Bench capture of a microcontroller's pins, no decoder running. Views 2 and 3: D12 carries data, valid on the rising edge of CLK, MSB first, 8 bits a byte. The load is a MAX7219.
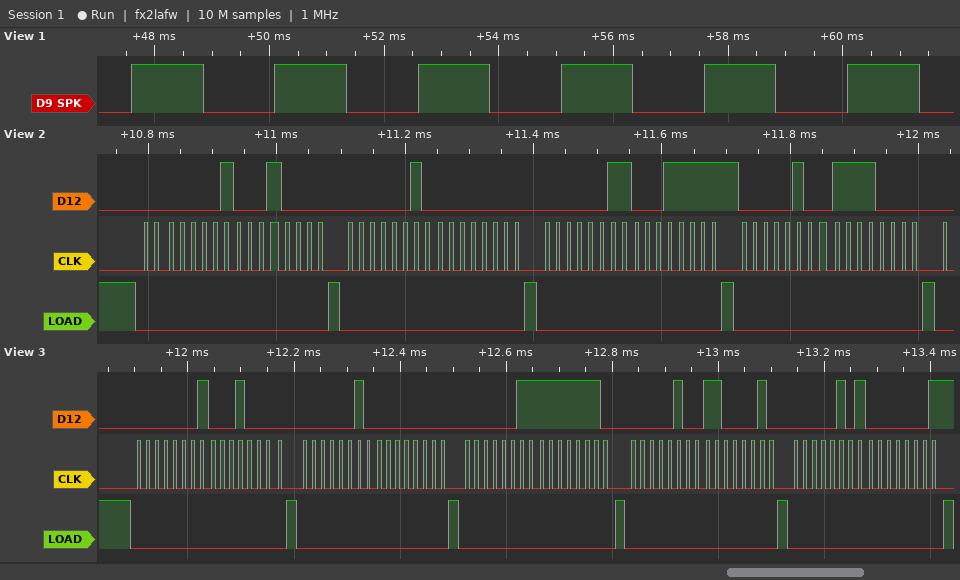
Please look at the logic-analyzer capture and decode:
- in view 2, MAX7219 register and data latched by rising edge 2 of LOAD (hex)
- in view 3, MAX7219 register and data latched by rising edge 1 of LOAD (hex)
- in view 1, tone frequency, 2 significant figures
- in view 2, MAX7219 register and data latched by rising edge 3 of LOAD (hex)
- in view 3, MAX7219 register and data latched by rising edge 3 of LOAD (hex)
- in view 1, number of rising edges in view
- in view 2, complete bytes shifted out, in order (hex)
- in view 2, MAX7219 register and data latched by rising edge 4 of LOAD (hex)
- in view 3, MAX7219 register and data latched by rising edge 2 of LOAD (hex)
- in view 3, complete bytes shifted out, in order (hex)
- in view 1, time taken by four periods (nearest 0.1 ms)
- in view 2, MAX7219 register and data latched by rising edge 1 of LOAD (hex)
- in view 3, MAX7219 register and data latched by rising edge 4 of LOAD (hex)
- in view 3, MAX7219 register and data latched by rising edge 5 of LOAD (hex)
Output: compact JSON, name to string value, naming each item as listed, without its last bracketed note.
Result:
{"in view 2, MAX7219 register and data latched by rising edge 2 of LOAD": "register 0x2, data 0x00", "in view 3, MAX7219 register and data latched by rising edge 1 of LOAD": "register 0x1, data 0x10", "in view 1, tone frequency, 2 significant figures": "400 Hz", "in view 2, MAX7219 register and data latched by rising edge 3 of LOAD": "register 0x3, data 0x1F", "in view 3, MAX7219 register and data latched by rising edge 3 of LOAD": "register 0x3, data 0xFE", "in view 1, number of rising edges in view": "6", "in view 2, complete bytes shifted out, in order": "01 10 02 00 03 1F 04 F0", "in view 2, MAX7219 register and data latched by rising edge 4 of LOAD": "register 0x4, data 0xF0", "in view 3, MAX7219 register and data latched by rising edge 2 of LOAD": "register 0x2, data 0x00", "in view 3, complete bytes shifted out, in order": "01 10 02 00 03 FE 04 C2 05 01", "in view 1, time taken by four periods": "10.0 ms", "in view 2, MAX7219 register and data latched by rising edge 1 of LOAD": "register 0x1, data 0x10", "in view 3, MAX7219 register and data latched by rising edge 4 of LOAD": "register 0x4, data 0xC2", "in view 3, MAX7219 register and data latched by rising edge 5 of LOAD": "register 0x5, data 0x01"}
